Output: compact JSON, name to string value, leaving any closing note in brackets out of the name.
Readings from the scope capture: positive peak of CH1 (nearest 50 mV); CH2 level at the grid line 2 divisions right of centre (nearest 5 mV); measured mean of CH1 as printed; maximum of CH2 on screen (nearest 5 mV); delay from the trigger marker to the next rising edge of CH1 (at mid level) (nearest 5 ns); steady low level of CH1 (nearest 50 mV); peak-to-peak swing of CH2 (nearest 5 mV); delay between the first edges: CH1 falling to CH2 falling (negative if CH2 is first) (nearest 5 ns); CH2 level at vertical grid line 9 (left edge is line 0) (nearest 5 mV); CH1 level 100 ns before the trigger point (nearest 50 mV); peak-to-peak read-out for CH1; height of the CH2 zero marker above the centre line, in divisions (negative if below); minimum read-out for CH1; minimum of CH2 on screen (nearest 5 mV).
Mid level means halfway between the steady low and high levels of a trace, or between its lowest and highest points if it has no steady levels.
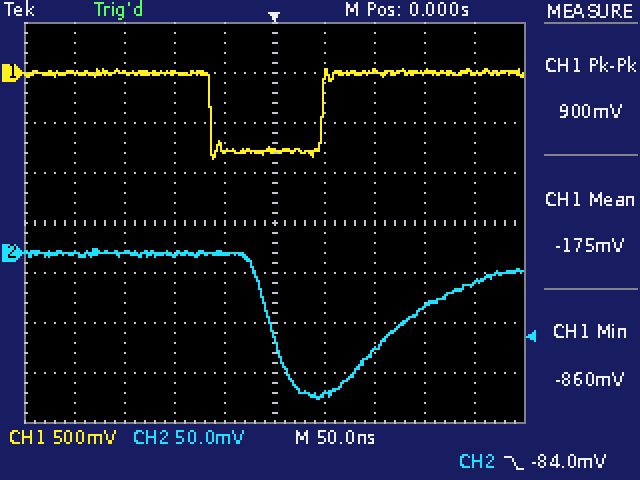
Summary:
{"positive peak of CH1": "50 mV", "CH2 level at the grid line 2 divisions right of centre": "-100 mV", "measured mean of CH1 as printed": "-175 mV", "maximum of CH2 on screen": "5 mV", "delay from the trigger marker to the next rising edge of CH1 (at mid level)": "50 ns", "steady low level of CH1": "-800 mV", "peak-to-peak swing of CH2": "150 mV", "delay between the first edges: CH1 falling to CH2 falling (negative if CH2 is first)": "+60 ns", "CH2 level at vertical grid line 9 (left edge is line 0)": "-30 mV", "CH1 level 100 ns before the trigger point": "0 mV", "peak-to-peak read-out for CH1": "900 mV", "height of the CH2 zero marker above the centre line, in divisions": "-0.6 div", "minimum read-out for CH1": "-860 mV", "minimum of CH2 on screen": "-145 mV"}
